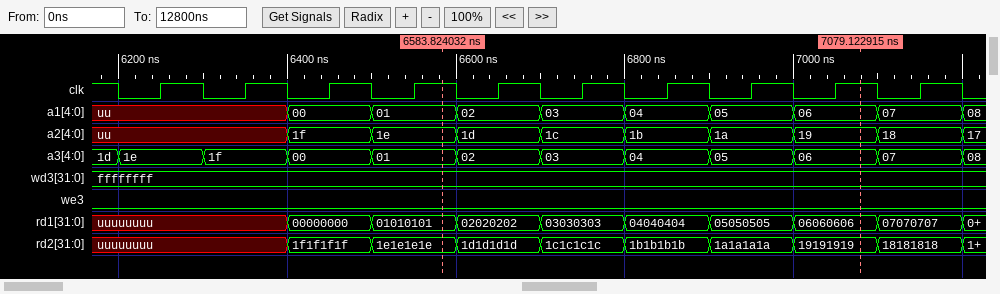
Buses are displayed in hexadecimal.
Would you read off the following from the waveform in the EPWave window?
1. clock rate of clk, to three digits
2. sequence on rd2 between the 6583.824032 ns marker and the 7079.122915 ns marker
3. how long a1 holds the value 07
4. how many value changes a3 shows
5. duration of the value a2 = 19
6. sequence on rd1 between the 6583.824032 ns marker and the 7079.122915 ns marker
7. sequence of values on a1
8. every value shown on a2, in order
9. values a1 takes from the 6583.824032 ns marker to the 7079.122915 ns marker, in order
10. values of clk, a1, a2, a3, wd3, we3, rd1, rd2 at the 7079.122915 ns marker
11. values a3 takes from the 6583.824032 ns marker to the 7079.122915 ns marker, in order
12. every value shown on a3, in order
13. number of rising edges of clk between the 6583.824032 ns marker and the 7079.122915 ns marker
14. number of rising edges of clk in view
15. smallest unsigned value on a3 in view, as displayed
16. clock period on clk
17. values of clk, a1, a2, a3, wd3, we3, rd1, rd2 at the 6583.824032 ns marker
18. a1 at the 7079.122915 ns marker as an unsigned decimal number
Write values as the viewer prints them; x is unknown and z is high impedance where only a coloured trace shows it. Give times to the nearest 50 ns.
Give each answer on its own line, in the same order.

10.0 MHz
1e1e1e1e, 1d1d1d1d, 1c1c1c1c, 1b1b1b1b, 1a1a1a1a, 19191919
100 ns
11
100 ns
01010101, 02020202, 03030303, 04040404, 05050505, 06060606
uu, 00, 01, 02, 03, 04, 05, 06, 07, 08
uu, 1f, 1e, 1d, 1c, 1b, 1a, 19, 18, 17
01, 02, 03, 04, 05, 06
clk=1, a1=06, a2=19, a3=06, wd3=ffffffff, we3=0, rd1=06060606, rd2=19191919
01, 02, 03, 04, 05, 06
1d, 1e, 1f, 00, 01, 02, 03, 04, 05, 06, 07, 08
5
10
00
100 ns
clk=1, a1=01, a2=1e, a3=01, wd3=ffffffff, we3=0, rd1=01010101, rd2=1e1e1e1e
6
